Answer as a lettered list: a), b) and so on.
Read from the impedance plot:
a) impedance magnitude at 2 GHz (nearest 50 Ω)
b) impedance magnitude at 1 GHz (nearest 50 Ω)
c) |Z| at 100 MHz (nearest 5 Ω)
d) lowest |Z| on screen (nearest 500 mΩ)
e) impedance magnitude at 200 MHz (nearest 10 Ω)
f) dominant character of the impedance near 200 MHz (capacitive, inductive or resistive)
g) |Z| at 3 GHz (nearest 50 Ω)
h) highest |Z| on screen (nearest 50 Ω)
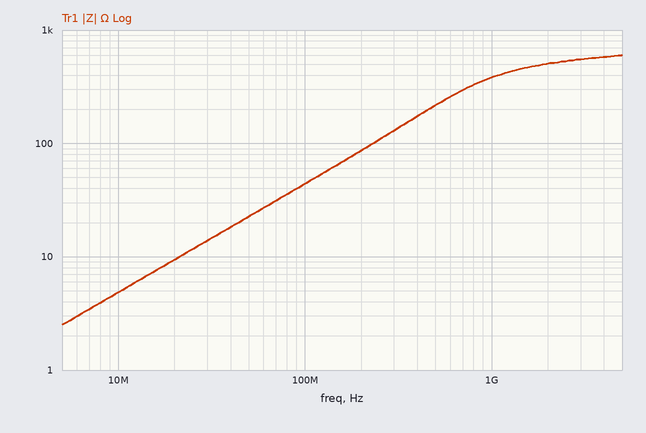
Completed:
a) 500 Ω
b) 400 Ω
c) 45 Ω
d) 2.5 Ω
e) 90 Ω
f) inductive
g) 550 Ω
h) 600 Ω
